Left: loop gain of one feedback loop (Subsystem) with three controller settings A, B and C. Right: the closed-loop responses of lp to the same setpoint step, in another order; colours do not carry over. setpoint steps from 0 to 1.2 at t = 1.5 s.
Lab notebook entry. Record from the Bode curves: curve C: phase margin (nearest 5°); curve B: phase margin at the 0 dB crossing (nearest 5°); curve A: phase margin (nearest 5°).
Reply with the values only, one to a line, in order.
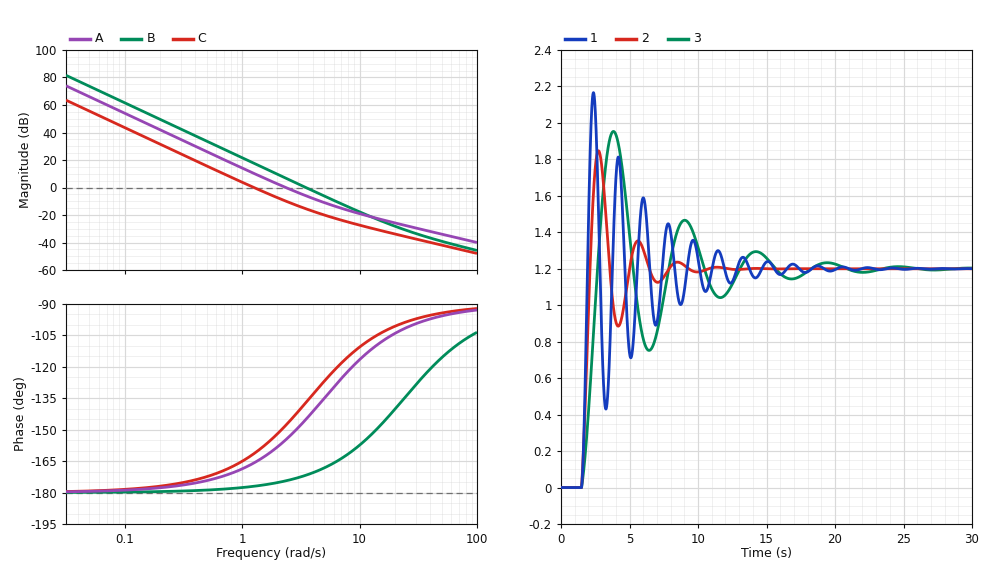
20°
10°
25°
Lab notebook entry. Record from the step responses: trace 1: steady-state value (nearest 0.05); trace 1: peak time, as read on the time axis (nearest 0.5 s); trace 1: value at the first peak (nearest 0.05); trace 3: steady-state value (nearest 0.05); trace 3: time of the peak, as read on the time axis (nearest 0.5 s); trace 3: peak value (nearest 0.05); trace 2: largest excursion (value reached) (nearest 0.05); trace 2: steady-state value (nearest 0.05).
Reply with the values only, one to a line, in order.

1.20
2.5 s
2.15
1.20
4.0 s
1.95
1.85
1.20
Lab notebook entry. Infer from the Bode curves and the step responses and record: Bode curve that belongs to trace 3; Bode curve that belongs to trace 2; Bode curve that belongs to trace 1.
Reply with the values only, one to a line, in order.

C
A
B
